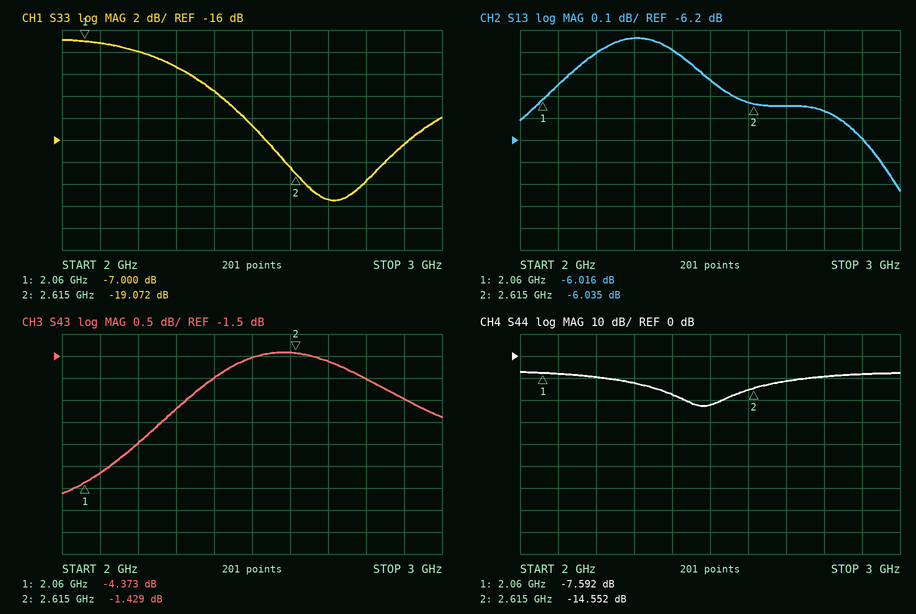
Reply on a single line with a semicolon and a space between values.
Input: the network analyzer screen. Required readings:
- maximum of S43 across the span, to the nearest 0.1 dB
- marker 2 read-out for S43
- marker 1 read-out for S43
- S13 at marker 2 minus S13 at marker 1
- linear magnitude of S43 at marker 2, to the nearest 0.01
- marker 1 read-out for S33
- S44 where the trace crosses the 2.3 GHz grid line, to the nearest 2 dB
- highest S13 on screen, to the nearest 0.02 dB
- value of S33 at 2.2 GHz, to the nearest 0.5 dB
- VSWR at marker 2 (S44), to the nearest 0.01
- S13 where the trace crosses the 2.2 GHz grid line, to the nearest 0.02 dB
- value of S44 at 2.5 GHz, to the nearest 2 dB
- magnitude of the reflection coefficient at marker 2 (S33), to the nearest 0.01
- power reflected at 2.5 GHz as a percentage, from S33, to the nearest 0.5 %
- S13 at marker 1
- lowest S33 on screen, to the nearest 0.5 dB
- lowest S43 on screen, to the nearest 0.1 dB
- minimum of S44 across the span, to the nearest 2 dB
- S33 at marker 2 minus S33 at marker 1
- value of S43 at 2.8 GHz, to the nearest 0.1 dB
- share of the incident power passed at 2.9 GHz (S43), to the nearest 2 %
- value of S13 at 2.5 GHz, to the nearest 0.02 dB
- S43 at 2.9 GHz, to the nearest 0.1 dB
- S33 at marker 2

-1.4 dB; -1.429 dB; -4.373 dB; -0.019 dB; 0.85; -7.000 dB; -12 dB; -5.74 dB; -8.0 dB; 1.46; -5.80 dB; -22 dB; 0.11; 3.5 %; -6.016 dB; -21.5 dB; -4.6 dB; -22 dB; -12.072 dB; -2.0 dB; 56 %; -5.92 dB; -2.5 dB; -19.072 dB
